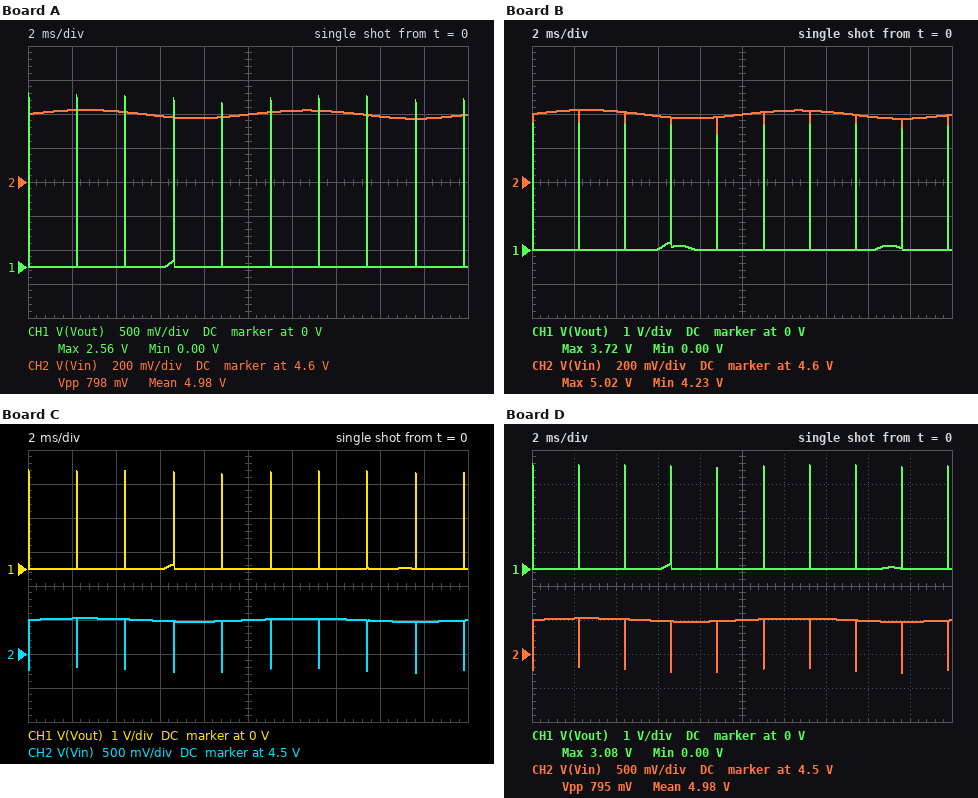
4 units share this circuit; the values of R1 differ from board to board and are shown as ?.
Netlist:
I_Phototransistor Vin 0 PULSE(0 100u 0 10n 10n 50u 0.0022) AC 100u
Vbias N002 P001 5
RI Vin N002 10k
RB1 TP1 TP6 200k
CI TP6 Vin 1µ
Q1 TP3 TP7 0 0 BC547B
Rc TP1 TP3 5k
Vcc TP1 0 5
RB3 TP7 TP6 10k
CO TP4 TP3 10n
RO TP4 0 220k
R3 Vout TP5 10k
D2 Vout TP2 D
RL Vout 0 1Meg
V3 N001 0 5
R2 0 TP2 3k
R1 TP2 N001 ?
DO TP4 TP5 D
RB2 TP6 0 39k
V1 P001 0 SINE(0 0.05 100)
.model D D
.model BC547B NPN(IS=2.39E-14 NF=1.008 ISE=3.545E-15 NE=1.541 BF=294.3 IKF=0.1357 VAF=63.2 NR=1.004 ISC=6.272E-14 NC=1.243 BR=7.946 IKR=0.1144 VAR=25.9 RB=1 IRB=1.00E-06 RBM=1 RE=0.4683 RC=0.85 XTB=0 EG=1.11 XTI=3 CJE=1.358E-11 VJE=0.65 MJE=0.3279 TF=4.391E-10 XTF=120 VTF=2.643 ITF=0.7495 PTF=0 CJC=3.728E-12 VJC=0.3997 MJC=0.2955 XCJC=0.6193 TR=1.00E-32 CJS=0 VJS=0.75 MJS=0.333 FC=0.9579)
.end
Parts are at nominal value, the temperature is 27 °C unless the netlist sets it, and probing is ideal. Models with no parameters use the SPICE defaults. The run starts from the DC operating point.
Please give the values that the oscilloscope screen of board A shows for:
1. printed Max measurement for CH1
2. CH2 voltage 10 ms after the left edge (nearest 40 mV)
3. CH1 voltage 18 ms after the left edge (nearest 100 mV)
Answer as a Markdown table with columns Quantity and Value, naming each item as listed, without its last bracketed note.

| Quantity | Value |
|---|---|
| printed Max measurement for CH1 | 2.56 V |
| CH2 voltage 10 ms after the left edge | 5.00 V |
| CH1 voltage 18 ms after the left edge | 0 V |
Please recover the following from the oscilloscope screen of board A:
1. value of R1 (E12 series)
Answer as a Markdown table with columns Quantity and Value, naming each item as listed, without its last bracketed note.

| Quantity | Value |
|---|---|
| value of R1 | 5.6 kΩ |
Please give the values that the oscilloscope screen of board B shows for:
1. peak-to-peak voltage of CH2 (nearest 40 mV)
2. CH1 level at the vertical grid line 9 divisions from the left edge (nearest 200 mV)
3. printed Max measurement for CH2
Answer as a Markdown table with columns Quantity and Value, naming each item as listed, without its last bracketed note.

| Quantity | Value |
|---|---|
| peak-to-peak voltage of CH2 | 800 mV |
| CH1 level at the vertical grid line 9 divisions from the left edge | 0 V |
| printed Max measurement for CH2 | 5.02 V |
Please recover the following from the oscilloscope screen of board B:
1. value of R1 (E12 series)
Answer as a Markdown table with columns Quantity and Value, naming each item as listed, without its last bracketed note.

| Quantity | Value |
|---|---|
| value of R1 | 1.8 kΩ |
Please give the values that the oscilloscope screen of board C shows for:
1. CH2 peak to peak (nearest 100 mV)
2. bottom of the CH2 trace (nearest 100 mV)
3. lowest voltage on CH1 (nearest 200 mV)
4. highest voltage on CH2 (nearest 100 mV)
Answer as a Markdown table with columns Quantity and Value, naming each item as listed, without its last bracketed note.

| Quantity | Value |
|---|---|
| CH2 peak to peak | 800 mV |
| bottom of the CH2 trace | 4.2 V |
| lowest voltage on CH1 | 0 V |
| highest voltage on CH2 | 5.0 V |
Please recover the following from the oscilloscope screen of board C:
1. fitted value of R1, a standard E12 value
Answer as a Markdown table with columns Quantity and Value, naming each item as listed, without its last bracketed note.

| Quantity | Value |
|---|---|
| fitted value of R1, a standard E12 value | 3.9 kΩ |
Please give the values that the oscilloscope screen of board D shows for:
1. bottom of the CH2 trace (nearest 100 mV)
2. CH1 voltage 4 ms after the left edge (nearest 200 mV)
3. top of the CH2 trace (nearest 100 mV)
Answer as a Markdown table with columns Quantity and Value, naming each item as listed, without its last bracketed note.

| Quantity | Value |
|---|---|
| bottom of the CH2 trace | 4.2 V |
| CH1 voltage 4 ms after the left edge | 0 V |
| top of the CH2 trace | 5.0 V |
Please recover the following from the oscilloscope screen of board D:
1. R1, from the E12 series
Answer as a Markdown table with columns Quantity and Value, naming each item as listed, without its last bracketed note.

| Quantity | Value |
|---|---|
| R1, from the E12 series | 3.3 kΩ |
